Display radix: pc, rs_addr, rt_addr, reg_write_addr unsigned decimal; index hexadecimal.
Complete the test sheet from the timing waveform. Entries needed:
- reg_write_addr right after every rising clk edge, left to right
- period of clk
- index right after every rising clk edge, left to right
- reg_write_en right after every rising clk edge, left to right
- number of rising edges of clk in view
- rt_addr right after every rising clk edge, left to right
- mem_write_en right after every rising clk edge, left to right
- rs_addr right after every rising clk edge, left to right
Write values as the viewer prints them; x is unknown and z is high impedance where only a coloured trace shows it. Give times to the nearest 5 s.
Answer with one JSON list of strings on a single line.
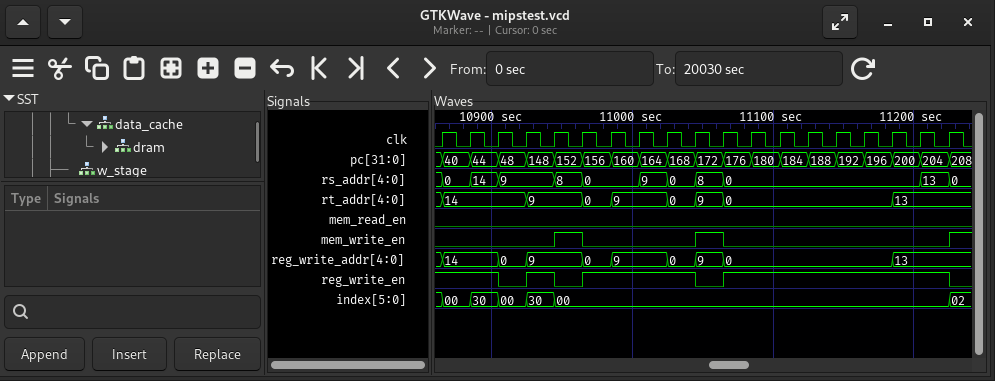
["14, 14, 0, 9, 9, 0, 9, 9, 0, 9, 0, 0, 0, 0, 0, 0, 13, 13, 13", "20 s", "00, 30, 00, 30, 00, 00, 00, 00, 00, 00, 00, 00, 00, 00, 00, 00, 00, 00, 02", "1 1 0 1 0 1 1 1 1 0 1 1 1 1 1 1 1 1 0", "19", "14, 14, 14, 9, 9, 0, 9, 9, 0, 9, 0, 0, 0, 0, 0, 0, 13, 13, 13", "0 0 0 0 1 0 0 0 0 1 0 0 0 0 0 0 0 0 1", "0, 14, 9, 9, 8, 0, 0, 9, 0, 8, 0, 0, 0, 0, 0, 0, 0, 13, 0"]
